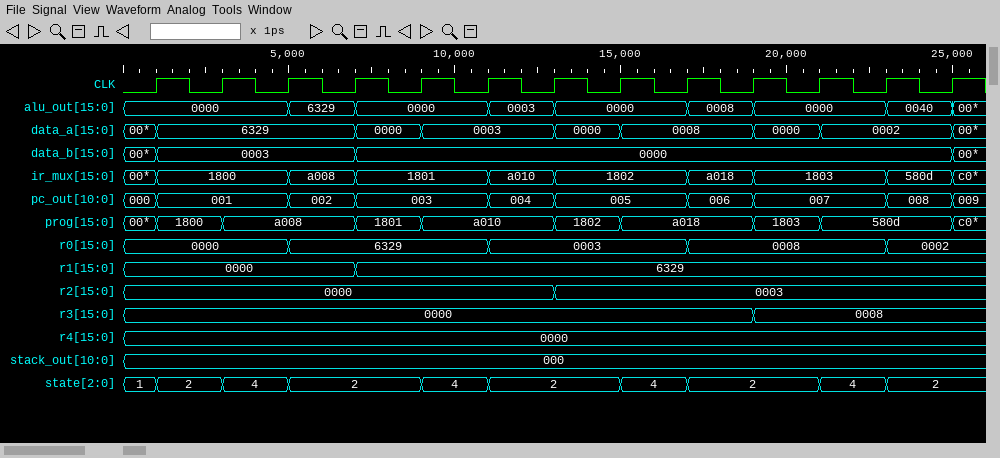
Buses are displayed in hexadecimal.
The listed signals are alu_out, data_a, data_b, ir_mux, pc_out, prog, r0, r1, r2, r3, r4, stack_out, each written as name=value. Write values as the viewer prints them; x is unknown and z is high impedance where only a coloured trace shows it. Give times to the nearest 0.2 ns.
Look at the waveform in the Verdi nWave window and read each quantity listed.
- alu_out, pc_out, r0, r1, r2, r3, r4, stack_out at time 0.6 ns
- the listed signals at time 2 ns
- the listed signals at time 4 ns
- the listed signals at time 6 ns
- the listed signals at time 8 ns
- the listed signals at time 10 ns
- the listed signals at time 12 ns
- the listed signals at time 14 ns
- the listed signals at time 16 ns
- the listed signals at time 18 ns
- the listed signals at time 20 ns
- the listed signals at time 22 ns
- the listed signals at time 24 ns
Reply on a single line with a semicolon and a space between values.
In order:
alu_out=0000, pc_out=000, r0=0000, r1=0000, r2=0000, r3=0000, r4=0000, stack_out=000; alu_out=0000, data_a=6329, data_b=0003, ir_mux=1800, pc_out=001, prog=1800, r0=0000, r1=0000, r2=0000, r3=0000, r4=0000, stack_out=000; alu_out=0000, data_a=6329, data_b=0003, ir_mux=1800, pc_out=001, prog=a008, r0=0000, r1=0000, r2=0000, r3=0000, r4=0000, stack_out=000; alu_out=6329, data_a=6329, data_b=0003, ir_mux=a008, pc_out=002, prog=a008, r0=6329, r1=0000, r2=0000, r3=0000, r4=0000, stack_out=000; alu_out=0000, data_a=0000, data_b=0000, ir_mux=1801, pc_out=003, prog=1801, r0=6329, r1=6329, r2=0000, r3=0000, r4=0000, stack_out=000; alu_out=0000, data_a=0003, data_b=0000, ir_mux=1801, pc_out=003, prog=a010, r0=6329, r1=6329, r2=0000, r3=0000, r4=0000, stack_out=000; alu_out=0003, data_a=0003, data_b=0000, ir_mux=a010, pc_out=004, prog=a010, r0=0003, r1=6329, r2=0000, r3=0000, r4=0000, stack_out=000; alu_out=0000, data_a=0000, data_b=0000, ir_mux=1802, pc_out=005, prog=1802, r0=0003, r1=6329, r2=0003, r3=0000, r4=0000, stack_out=000; alu_out=0000, data_a=0008, data_b=0000, ir_mux=1802, pc_out=005, prog=a018, r0=0003, r1=6329, r2=0003, r3=0000, r4=0000, stack_out=000; alu_out=0008, data_a=0008, data_b=0000, ir_mux=a018, pc_out=006, prog=a018, r0=0008, r1=6329, r2=0003, r3=0000, r4=0000, stack_out=000; alu_out=0000, data_a=0000, data_b=0000, ir_mux=1803, pc_out=007, prog=1803, r0=0008, r1=6329, r2=0003, r3=0008, r4=0000, stack_out=000; alu_out=0000, data_a=0002, data_b=0000, ir_mux=1803, pc_out=007, prog=580d, r0=0008, r1=6329, r2=0003, r3=0008, r4=0000, stack_out=000; alu_out=0040, data_a=0002, data_b=0000, ir_mux=580d, pc_out=008, prog=580d, r0=0002, r1=6329, r2=0003, r3=0008, r4=0000, stack_out=000
